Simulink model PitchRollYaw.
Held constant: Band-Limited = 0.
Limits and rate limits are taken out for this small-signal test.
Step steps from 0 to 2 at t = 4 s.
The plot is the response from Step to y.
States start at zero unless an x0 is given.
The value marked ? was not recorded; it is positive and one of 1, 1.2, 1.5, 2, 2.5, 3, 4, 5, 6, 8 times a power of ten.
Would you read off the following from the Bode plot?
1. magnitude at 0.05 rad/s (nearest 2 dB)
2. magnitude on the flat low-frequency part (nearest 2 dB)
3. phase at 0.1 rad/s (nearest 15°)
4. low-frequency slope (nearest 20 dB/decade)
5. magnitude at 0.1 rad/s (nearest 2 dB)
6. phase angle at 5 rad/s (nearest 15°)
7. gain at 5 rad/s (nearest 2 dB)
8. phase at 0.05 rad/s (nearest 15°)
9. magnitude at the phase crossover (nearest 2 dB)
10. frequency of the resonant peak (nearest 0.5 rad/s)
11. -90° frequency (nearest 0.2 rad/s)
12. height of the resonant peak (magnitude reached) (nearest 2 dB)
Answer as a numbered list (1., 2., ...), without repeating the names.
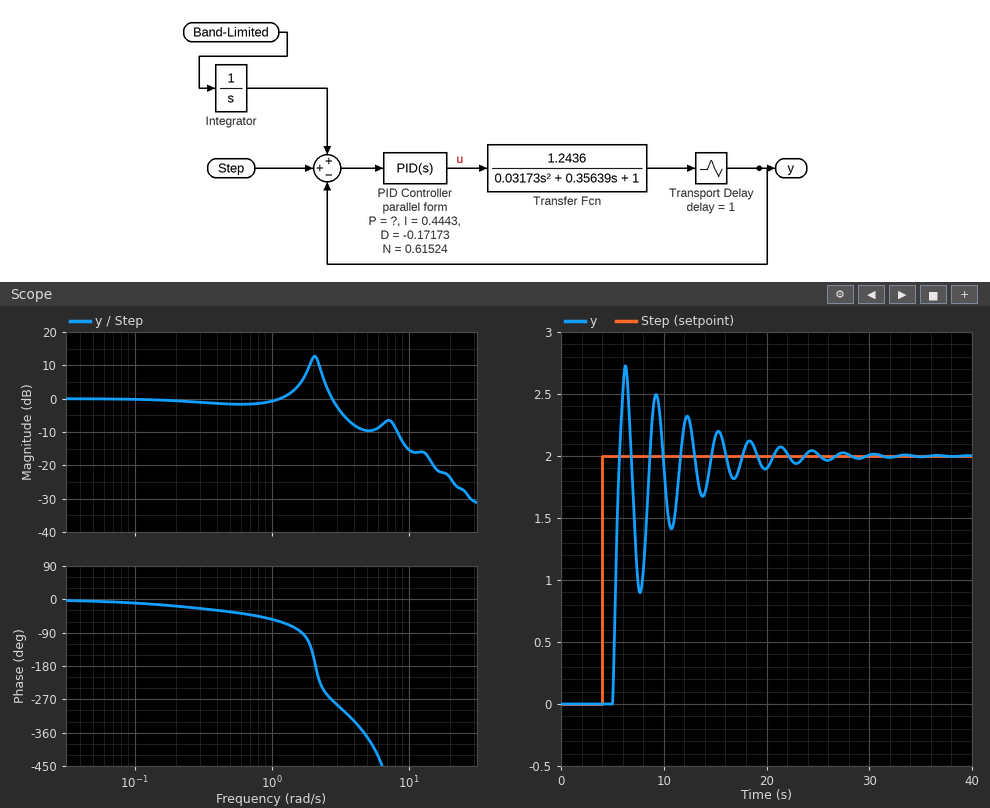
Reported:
1. 0 dB
2. 0 dB
3. -15°
4. 0 dB/decade
5. 0 dB
6. -375°
7. -10 dB
8. 0°
9. 12 dB
10. 2.0 rad/s
11. 1.6 rad/s
12. 12 dB
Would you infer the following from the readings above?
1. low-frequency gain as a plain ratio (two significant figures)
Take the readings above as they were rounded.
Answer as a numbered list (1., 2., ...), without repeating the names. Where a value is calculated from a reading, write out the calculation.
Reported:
1. 10^(0 / 20) = 1.0
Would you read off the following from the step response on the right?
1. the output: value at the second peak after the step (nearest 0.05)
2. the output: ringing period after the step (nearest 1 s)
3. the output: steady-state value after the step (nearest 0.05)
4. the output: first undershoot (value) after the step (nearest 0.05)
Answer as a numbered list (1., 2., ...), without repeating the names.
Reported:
1. 2.50
2. 3 s
3. 2.00
4. 0.90
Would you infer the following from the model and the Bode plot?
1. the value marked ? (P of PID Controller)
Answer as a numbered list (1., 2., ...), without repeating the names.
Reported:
1. 0.8
